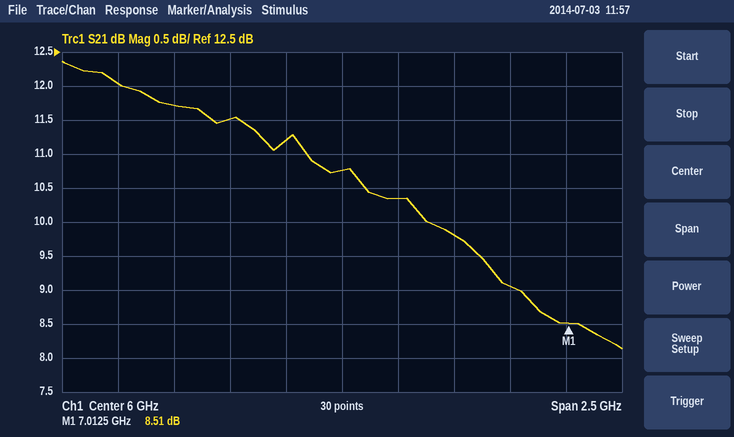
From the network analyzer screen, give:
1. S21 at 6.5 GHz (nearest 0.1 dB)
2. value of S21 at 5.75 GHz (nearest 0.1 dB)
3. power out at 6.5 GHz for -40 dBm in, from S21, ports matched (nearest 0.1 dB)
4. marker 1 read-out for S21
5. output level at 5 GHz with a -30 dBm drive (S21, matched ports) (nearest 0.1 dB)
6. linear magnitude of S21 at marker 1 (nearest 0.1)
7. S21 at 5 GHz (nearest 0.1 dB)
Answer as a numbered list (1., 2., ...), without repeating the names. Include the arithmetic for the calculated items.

1. 9.8 dB
2. 11.2 dB
3. -40 dBm + (9.8 dB) = -30.2 dBm
4. 8.51 dB
5. -30 dBm + (12.0 dB) = -18.0 dBm
6. 10^(8.51/20) ≈ 2.7
7. 12.0 dB
